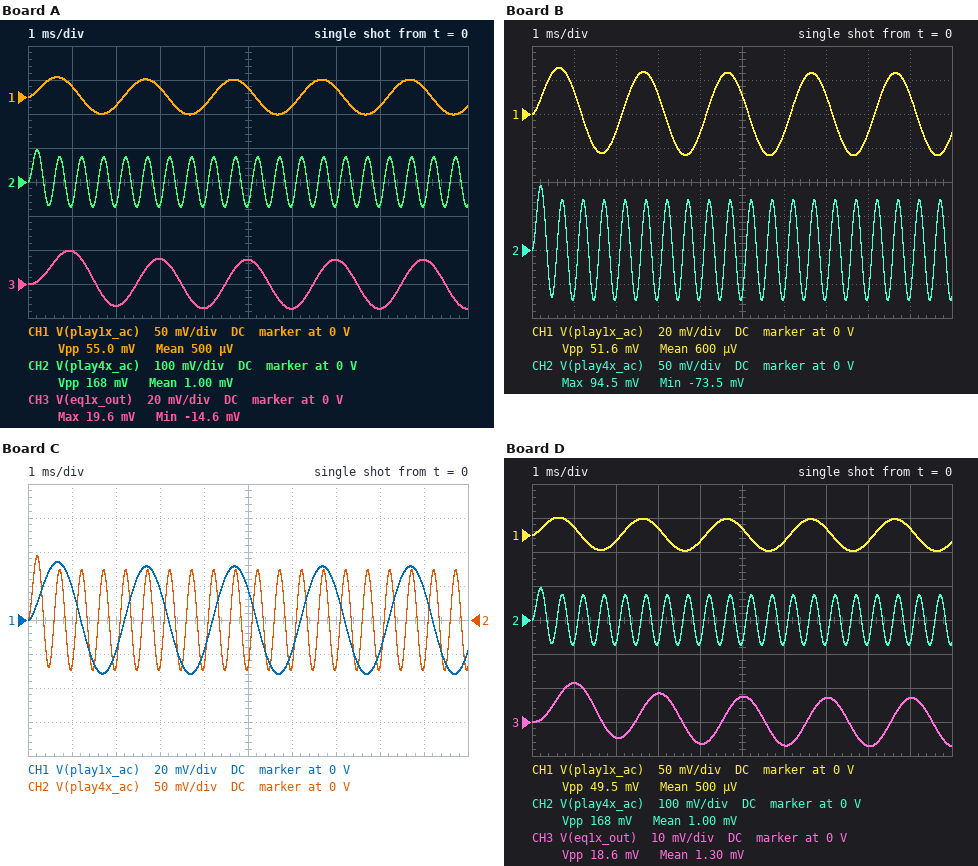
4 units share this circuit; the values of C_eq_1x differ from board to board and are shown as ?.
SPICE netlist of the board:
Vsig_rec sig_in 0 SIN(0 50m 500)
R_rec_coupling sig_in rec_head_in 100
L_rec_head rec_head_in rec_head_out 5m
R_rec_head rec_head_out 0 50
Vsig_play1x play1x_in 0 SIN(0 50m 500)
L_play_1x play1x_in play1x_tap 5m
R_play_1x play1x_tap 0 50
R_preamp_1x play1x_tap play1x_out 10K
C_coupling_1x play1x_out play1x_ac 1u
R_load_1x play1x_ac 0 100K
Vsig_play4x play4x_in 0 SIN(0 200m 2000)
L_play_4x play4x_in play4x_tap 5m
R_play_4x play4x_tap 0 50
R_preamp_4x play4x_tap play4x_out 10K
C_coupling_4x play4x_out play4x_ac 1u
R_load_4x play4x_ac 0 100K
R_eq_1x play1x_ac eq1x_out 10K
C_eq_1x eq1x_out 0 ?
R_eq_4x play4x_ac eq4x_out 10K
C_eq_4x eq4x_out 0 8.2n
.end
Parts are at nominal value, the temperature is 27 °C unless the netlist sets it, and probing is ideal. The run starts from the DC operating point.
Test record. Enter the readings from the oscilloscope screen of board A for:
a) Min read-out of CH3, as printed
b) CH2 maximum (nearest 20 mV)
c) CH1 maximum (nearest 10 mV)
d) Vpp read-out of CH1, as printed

-14.6 mV
100 mV
30 mV
55.0 mV
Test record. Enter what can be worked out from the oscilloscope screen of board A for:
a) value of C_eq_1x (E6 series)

47 nF
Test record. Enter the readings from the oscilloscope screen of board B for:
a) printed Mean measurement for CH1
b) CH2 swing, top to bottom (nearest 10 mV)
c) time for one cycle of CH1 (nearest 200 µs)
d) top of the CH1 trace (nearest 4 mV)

600 µV
170 mV
2.0 ms
28 mV
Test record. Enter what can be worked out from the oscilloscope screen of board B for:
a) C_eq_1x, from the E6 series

68 nF
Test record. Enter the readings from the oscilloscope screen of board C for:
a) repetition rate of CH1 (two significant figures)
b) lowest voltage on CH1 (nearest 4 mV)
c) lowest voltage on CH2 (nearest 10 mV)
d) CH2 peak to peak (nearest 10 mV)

500 Hz
-32 mV
-70 mV
170 mV
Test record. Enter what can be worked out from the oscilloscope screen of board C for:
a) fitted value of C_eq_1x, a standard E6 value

22 nF
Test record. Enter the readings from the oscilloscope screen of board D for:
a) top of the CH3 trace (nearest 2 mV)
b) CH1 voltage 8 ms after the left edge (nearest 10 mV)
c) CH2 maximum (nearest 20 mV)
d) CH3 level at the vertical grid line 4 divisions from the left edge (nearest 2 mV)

12 mV
-10 mV
100 mV
-6 mV
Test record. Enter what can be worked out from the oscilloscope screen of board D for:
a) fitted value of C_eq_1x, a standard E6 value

100 nF
